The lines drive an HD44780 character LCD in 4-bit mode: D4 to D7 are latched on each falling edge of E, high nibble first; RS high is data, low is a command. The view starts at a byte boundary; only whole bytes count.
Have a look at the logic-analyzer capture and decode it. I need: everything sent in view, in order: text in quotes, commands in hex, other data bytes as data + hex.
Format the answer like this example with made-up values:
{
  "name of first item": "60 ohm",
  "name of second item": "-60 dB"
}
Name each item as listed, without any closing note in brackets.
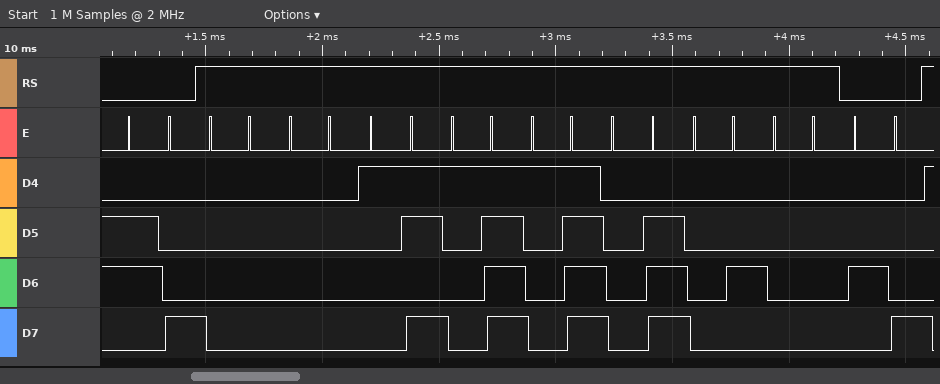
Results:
{
  "everything sent in view, in order: text in quotes, commands in hex, other data bytes as data + hex": "0x68 data 00 00 1B 1F 1F 0E 04 00 0x48"
}
